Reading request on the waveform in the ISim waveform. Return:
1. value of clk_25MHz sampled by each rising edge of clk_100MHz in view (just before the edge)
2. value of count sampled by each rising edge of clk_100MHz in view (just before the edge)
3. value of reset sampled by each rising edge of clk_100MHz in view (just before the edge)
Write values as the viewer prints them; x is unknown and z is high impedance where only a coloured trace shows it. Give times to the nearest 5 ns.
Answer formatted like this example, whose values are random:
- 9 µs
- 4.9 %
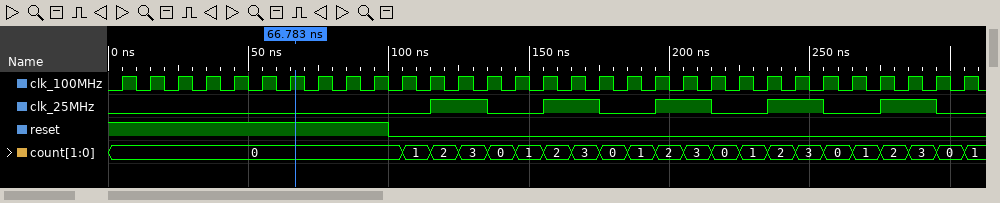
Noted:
- 0 0 0 0 0 0 0 0 0 0 0 0 1 1 0 0 1 1 0 0 1 1 0 0 1 1 0 0 1 1 0
- 0, 0, 0, 0, 0, 0, 0, 0, 0, 0, 0, 1, 2, 3, 0, 1, 2, 3, 0, 1, 2, 3, 0, 1, 2, 3, 0, 1, 2, 3, 0
- 1 1 1 1 1 1 1 1 1 1 0 0 0 0 0 0 0 0 0 0 0 0 0 0 0 0 0 0 0 0 0
